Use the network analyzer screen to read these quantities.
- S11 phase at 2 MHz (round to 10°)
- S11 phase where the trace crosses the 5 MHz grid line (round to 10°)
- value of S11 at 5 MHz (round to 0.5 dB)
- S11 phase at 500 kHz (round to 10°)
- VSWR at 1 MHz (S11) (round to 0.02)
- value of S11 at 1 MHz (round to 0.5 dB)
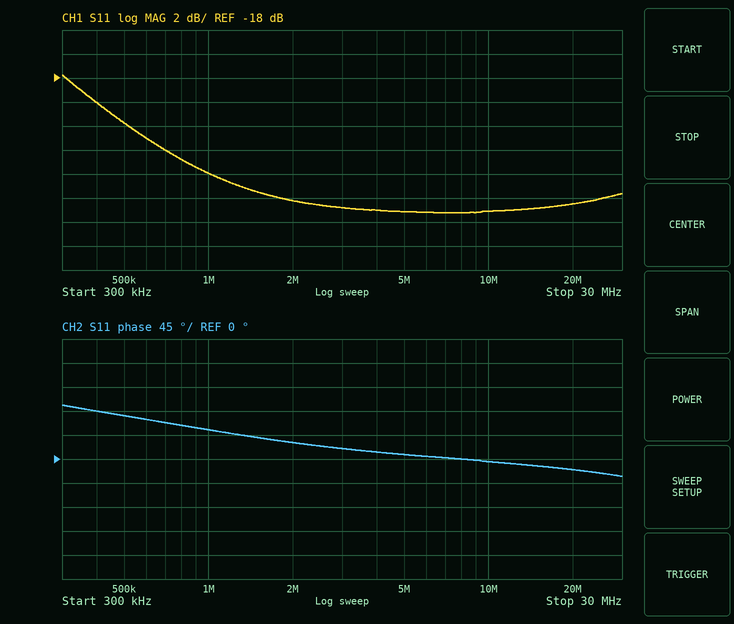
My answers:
30°
10°
-29.0 dB
80°
1.10
-26.0 dB
